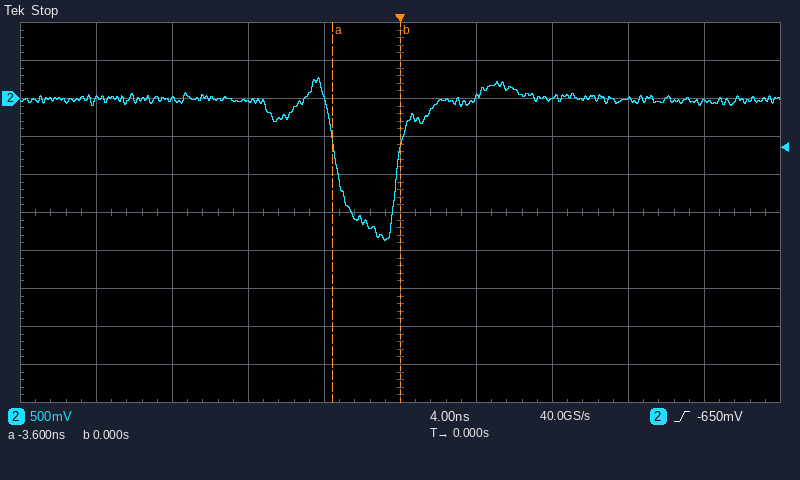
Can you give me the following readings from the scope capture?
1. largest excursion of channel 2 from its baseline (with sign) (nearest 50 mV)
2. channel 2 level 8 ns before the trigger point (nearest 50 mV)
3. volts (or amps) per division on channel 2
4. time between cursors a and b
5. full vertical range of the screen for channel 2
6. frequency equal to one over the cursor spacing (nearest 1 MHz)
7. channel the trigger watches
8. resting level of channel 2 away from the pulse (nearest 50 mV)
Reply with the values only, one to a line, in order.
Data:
-1.85 V
-50 mV
500 mV
3.6 ns
5 V
278 MHz
channel 2
0 mV
